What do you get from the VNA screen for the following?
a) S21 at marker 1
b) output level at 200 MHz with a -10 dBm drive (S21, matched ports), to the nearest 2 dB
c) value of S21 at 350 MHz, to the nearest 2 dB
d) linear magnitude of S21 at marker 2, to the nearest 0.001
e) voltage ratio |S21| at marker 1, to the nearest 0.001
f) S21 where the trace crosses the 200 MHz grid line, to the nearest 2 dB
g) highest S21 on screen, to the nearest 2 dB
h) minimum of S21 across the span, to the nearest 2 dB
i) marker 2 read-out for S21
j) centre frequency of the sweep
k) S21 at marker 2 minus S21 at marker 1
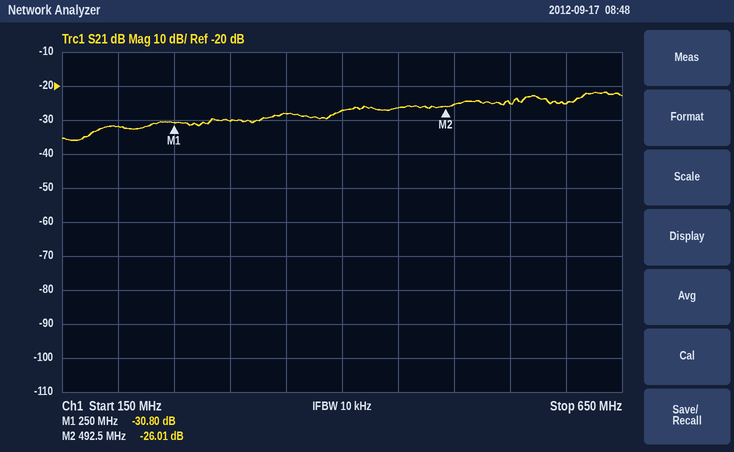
-30.80 dB
-42 dBm
-28 dB
0.050
0.029
-32 dB
-22 dB
-36 dB
-26.01 dB
400 MHz
4.79 dB
